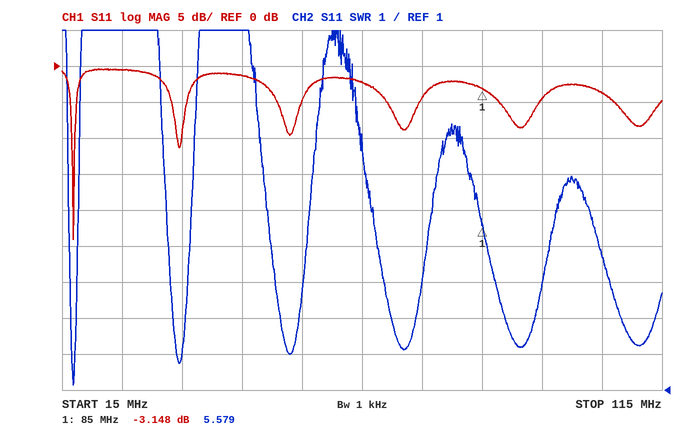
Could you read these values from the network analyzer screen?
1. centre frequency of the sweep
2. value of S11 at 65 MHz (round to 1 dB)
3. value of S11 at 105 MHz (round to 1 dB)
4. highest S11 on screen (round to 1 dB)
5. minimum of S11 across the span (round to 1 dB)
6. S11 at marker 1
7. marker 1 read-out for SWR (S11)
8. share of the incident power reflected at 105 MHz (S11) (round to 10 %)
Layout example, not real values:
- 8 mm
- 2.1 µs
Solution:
- 65 MHz
- -2 dB
- -4 dB
- 0 dB
- -24 dB
- -3.148 dB
- 5.579
- 40 %
